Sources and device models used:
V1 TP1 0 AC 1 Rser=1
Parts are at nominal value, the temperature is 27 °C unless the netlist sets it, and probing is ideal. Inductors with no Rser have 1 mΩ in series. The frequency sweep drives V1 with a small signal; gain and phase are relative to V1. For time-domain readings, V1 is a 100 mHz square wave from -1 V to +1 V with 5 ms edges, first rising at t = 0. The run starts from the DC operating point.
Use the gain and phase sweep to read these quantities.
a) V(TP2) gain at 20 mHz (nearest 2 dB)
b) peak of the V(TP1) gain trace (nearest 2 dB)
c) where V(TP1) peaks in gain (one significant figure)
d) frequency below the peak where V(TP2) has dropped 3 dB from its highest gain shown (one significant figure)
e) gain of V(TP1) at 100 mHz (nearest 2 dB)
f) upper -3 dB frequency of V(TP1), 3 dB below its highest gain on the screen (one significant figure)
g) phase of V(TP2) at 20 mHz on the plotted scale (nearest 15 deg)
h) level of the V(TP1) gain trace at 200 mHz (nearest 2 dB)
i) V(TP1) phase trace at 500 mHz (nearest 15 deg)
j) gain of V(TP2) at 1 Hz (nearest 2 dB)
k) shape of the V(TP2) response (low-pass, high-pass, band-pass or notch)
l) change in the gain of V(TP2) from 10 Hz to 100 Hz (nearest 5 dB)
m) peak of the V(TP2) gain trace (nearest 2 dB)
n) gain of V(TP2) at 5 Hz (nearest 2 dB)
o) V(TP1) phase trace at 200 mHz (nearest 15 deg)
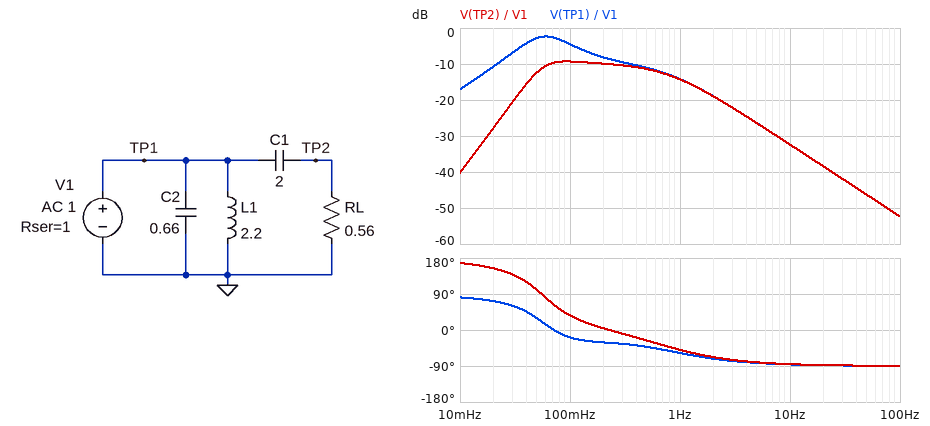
-28 dB
-2 dB
60 mHz
50 mHz
-4 dB
100 mHz
150 deg
-8 dB
-45 deg
-14 dB
band-pass
-20 dB
-10 dB
-26 dB
-30 deg
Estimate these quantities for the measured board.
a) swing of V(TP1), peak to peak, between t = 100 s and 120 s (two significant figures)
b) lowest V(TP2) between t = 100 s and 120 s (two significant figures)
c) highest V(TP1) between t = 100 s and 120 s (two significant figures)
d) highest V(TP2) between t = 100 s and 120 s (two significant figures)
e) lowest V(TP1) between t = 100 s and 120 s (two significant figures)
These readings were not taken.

1.3 V
-570 mV
660 mV
570 mV
-660 mV
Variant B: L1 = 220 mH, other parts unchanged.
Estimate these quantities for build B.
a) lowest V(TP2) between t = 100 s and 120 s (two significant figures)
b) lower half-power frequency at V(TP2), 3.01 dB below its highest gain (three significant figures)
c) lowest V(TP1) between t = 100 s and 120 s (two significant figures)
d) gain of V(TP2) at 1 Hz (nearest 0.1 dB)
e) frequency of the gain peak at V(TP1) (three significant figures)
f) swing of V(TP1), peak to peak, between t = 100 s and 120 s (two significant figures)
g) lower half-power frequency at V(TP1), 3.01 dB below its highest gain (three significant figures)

-410 mV
188 mHz
-520 mV
-13.3 dB
308 mHz
1.0 V
162 mHz
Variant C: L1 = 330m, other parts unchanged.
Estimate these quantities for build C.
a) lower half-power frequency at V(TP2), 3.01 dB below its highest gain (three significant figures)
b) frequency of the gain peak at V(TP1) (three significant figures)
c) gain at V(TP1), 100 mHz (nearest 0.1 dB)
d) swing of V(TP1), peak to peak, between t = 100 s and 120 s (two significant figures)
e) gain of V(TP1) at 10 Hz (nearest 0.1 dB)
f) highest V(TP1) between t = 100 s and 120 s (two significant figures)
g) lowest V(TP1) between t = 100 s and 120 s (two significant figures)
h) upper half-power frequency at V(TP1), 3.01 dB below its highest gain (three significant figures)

142 mHz
210 mHz
-11.9 dB
1.2 V
-32.4 dB
590 mV
-590 mV
556 mHz
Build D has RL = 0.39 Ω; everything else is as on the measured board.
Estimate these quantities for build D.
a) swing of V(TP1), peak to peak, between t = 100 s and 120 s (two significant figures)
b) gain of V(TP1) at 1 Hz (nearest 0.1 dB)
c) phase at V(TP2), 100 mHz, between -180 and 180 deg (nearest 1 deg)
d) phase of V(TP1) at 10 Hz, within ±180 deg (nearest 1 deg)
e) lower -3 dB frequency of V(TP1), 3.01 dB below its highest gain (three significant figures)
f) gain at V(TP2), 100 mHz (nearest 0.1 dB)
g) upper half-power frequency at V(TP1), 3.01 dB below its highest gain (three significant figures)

1.4 V
-15.2 dB
39 deg
-85 deg
36.8 mHz
-11.5 dB
106 mHz
